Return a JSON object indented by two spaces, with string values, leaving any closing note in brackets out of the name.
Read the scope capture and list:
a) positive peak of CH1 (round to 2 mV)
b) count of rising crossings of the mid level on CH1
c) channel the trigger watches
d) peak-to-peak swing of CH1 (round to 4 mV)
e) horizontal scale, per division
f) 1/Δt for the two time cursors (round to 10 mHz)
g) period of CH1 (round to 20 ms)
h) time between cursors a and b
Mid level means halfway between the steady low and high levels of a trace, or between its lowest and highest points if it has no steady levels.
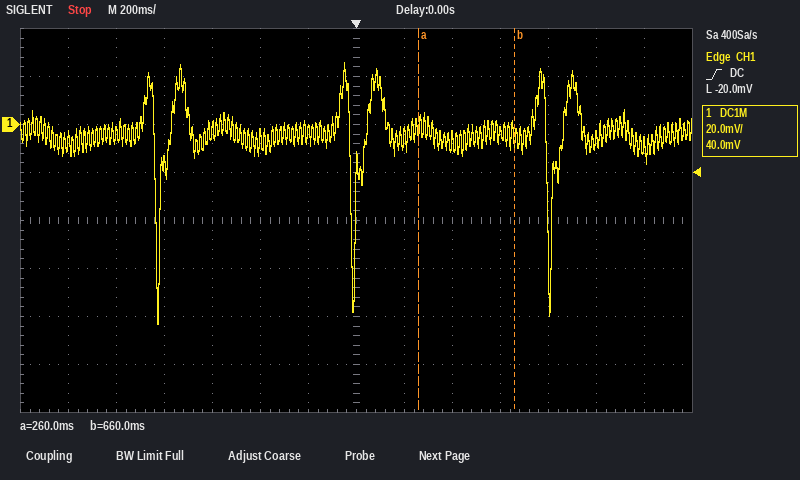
{
  "positive peak of CH1": "26 mV",
  "count of rising crossings of the mid level on CH1": "3",
  "channel the trigger watches": "CH1",
  "peak-to-peak swing of CH1": "108 mV",
  "horizontal scale, per division": "200 ms",
  "1/Δt for the two time cursors": "2.50 Hz",
  "period of CH1": "820 ms",
  "time between cursors a and b": "400 ms"
}
